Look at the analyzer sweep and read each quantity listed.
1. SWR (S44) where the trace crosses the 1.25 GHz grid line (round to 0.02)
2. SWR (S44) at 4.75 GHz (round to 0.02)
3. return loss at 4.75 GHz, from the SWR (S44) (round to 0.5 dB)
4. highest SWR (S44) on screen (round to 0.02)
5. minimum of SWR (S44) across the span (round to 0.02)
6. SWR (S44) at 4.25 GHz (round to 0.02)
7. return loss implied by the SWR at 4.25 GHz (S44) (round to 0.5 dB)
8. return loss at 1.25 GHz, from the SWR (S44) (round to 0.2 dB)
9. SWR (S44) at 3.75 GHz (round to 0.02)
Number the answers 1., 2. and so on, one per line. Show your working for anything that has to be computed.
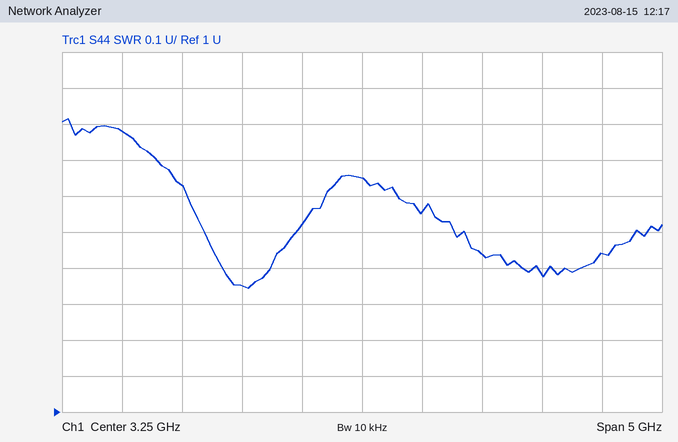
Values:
1. 1.78
2. 1.38
3. −20 log10((1.38 − 1)/(1.38 + 1)) ≈ 15.9 dB, so 16.0 dB to the nearest 0.5 dB
4. 1.82
5. 1.34
6. 1.44
7. −20 log10((1.44 − 1)/(1.44 + 1)) ≈ 14.9 dB, so 15.0 dB to the nearest 0.5 dB
8. −20 log10((1.78 − 1)/(1.78 + 1)) ≈ 11.0 dB
9. 1.56
